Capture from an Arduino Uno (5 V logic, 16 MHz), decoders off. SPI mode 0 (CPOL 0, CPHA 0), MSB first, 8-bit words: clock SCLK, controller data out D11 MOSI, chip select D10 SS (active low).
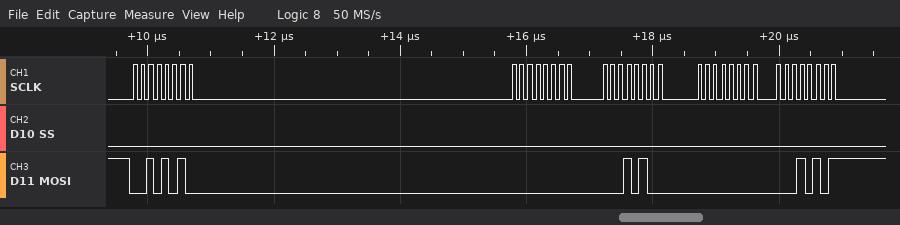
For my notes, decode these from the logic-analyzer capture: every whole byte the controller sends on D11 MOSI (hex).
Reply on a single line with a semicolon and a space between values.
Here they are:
2A 00 14 00 15
